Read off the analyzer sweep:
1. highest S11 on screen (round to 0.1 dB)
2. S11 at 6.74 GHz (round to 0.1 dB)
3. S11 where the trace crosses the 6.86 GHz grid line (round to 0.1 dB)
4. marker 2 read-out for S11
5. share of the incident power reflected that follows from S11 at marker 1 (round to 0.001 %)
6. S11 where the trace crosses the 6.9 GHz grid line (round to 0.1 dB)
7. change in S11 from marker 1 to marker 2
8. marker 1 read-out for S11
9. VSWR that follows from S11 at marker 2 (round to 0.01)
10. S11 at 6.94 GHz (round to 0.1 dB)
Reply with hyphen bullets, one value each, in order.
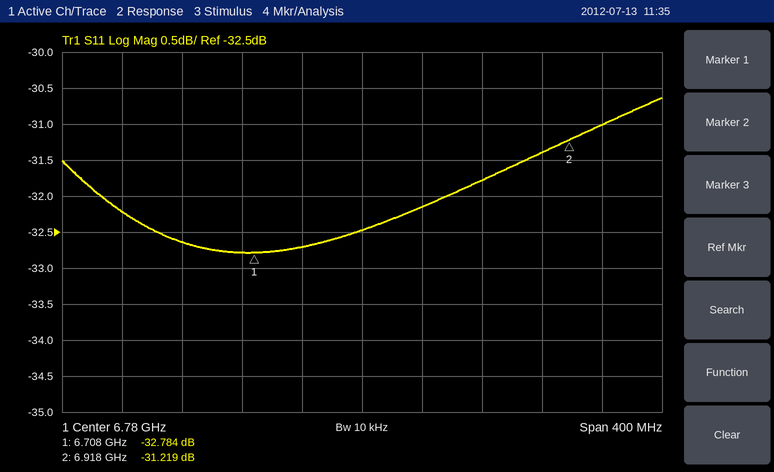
- -30.6 dB
- -32.7 dB
- -31.8 dB
- -31.219 dB
- 0.053 %
- -31.4 dB
- 1.565 dB
- -32.784 dB
- 1.06
- -31.0 dB
